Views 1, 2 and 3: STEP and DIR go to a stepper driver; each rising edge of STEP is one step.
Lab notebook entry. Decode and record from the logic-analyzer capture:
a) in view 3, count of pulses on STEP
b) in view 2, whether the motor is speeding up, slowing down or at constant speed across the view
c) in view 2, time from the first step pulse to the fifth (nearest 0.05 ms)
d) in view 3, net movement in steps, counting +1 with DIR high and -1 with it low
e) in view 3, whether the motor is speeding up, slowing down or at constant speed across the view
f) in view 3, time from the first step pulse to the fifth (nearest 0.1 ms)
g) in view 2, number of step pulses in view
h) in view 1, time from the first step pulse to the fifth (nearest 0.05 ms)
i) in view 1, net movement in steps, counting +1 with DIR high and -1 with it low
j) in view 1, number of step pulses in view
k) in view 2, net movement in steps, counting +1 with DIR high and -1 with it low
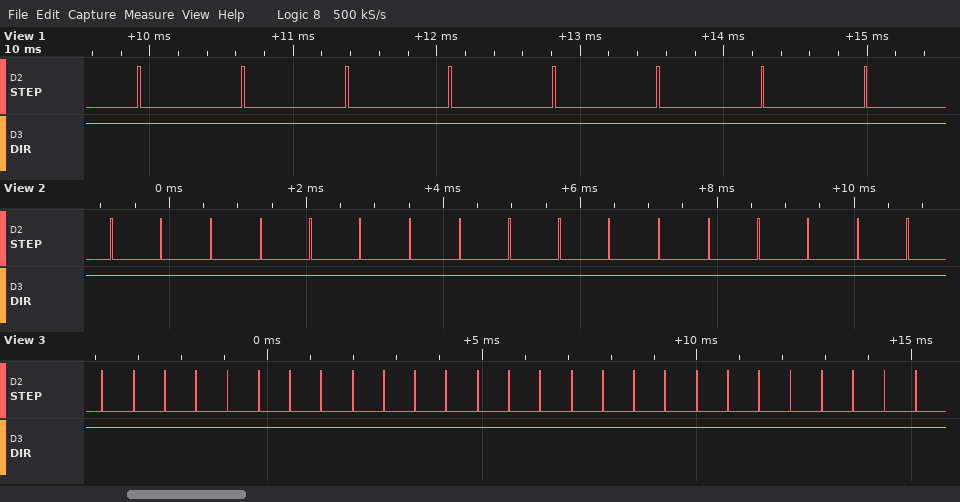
27
constant speed
2.90 ms
+27
constant speed
2.9 ms
17
2.90 ms
+8
8
+17
